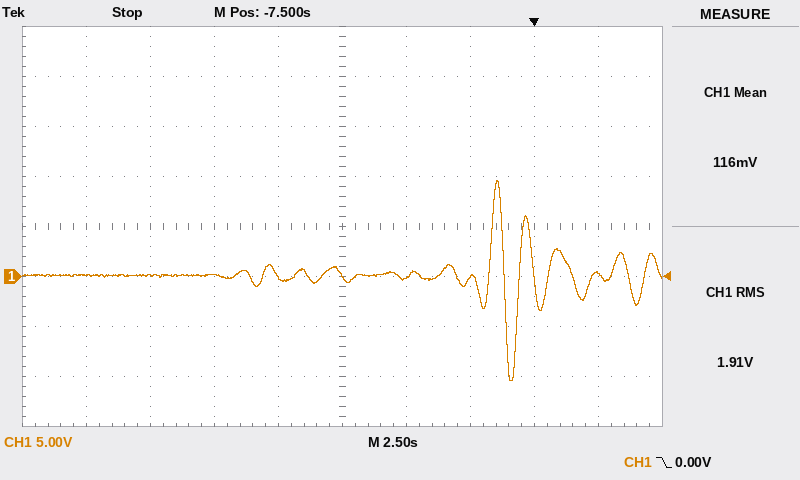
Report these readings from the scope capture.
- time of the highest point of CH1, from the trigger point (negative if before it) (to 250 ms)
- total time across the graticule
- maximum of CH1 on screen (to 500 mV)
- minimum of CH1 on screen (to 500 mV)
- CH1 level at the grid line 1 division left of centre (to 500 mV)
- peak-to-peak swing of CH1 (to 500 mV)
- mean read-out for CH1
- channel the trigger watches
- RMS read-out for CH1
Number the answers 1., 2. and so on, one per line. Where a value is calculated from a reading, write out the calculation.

1. -1.50 s
2. 25 s
3. 9.5 V
4. -10.5 V
5. 0.0 V
6. 9.5 V − (-10.5 V) = 20.0 V
7. 116 mV
8. CH1
9. 1.91 V
